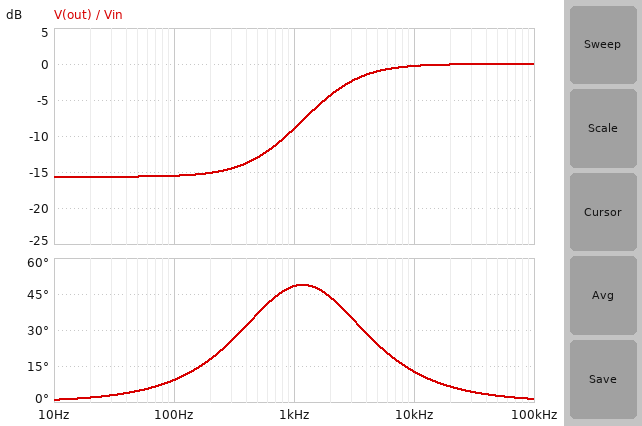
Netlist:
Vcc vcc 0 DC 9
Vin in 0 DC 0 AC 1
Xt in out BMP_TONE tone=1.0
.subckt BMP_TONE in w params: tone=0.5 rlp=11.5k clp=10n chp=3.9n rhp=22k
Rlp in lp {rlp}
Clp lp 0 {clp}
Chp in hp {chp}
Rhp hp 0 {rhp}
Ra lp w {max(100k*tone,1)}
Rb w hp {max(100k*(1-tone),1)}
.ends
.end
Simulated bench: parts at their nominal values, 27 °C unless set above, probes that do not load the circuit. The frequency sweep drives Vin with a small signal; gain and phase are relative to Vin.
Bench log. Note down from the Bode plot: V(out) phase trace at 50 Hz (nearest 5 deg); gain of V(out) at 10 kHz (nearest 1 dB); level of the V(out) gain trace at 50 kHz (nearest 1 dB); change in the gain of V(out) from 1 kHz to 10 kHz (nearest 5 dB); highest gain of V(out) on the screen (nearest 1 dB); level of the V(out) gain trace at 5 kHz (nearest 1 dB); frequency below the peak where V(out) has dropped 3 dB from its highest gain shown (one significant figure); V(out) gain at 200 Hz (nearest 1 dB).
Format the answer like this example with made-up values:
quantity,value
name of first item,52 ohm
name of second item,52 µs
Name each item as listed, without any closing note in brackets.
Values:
quantity,value
V(out) phase trace at 50 Hz,5 deg
gain of V(out) at 10 kHz,0 dB
level of the V(out) gain trace at 50 kHz,0 dB
change in the gain of V(out) from 1 kHz to 10 kHz,10 dB
highest gain of V(out) on the screen,0 dB
level of the V(out) gain trace at 5 kHz,-1 dB
frequency below the peak where V(out) has dropped 3 dB from its highest gain shown,3 kHz
V(out) gain at 200 Hz,-15 dB
